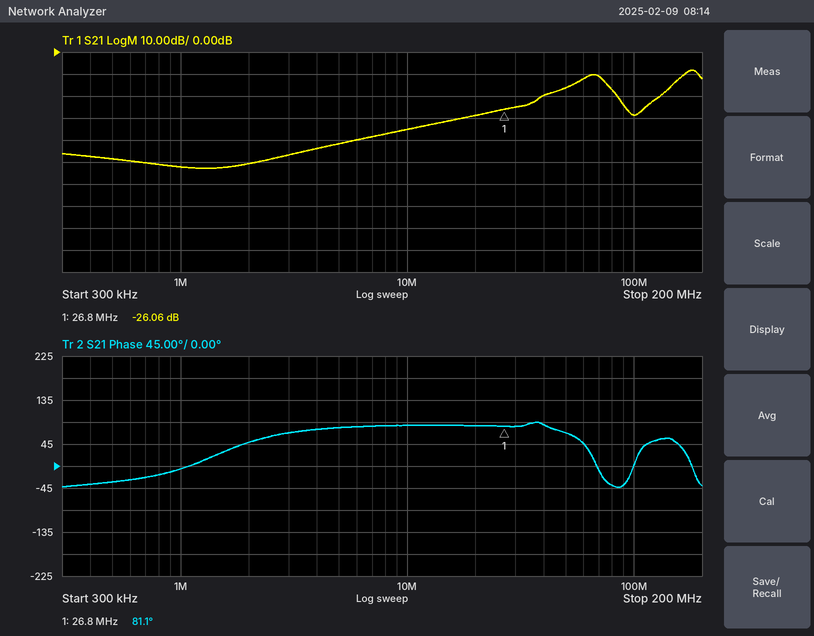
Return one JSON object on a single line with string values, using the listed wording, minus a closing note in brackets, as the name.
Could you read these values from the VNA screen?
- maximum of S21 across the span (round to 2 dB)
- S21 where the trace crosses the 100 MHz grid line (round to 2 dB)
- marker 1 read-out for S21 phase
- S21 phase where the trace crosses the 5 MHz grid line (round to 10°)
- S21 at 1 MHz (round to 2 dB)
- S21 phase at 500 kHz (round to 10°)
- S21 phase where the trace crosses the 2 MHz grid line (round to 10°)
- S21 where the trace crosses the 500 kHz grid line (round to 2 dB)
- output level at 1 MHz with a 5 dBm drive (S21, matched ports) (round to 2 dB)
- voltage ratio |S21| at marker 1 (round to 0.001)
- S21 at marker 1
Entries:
{"maximum of S21 across the span": "-8 dB", "S21 where the trace crosses the 100 MHz grid line": "-28 dB", "marker 1 read-out for S21 phase": "81.1°", "S21 phase where the trace crosses the 5 MHz grid line": "80°", "S21 at 1 MHz": "-52 dB", "S21 phase at 500 kHz": "-30°", "S21 phase where the trace crosses the 2 MHz grid line": "50°", "S21 where the trace crosses the 500 kHz grid line": "-48 dB", "output level at 1 MHz with a 5 dBm drive (S21, matched ports)": "-48 dBm", "voltage ratio |S21| at marker 1": "0.050", "S21 at marker 1": "-26.06 dB"}
